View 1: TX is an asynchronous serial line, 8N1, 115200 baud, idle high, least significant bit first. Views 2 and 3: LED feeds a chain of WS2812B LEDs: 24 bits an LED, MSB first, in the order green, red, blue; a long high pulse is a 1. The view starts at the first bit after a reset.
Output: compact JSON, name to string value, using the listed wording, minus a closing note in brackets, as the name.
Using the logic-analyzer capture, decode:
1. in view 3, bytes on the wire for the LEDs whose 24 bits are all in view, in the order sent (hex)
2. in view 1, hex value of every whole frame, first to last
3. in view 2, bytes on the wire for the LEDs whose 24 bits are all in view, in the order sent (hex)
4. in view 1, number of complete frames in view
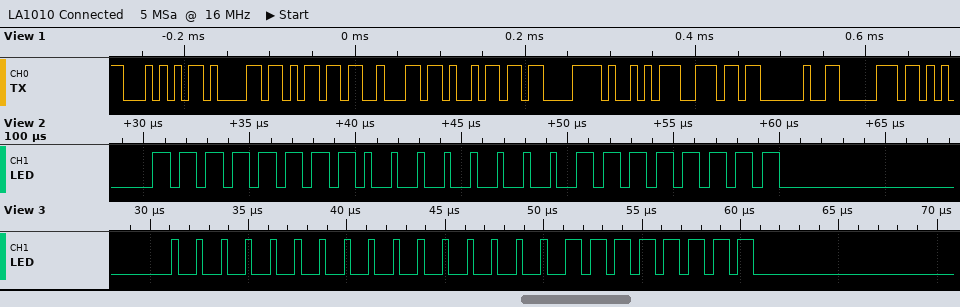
{"in view 3, bytes on the wire for the LEDs whose 24 bits are all in view, in the order sent": "00 00 FF", "in view 1, hex value of every whole frame, first to last": "54 61 6D 62 69 C3 A9 6E 20 70", "in view 2, bytes on the wire for the LEDs whose 24 bits are all in view, in the order sent": "FF 00 FF", "in view 1, number of complete frames in view": "10"}
